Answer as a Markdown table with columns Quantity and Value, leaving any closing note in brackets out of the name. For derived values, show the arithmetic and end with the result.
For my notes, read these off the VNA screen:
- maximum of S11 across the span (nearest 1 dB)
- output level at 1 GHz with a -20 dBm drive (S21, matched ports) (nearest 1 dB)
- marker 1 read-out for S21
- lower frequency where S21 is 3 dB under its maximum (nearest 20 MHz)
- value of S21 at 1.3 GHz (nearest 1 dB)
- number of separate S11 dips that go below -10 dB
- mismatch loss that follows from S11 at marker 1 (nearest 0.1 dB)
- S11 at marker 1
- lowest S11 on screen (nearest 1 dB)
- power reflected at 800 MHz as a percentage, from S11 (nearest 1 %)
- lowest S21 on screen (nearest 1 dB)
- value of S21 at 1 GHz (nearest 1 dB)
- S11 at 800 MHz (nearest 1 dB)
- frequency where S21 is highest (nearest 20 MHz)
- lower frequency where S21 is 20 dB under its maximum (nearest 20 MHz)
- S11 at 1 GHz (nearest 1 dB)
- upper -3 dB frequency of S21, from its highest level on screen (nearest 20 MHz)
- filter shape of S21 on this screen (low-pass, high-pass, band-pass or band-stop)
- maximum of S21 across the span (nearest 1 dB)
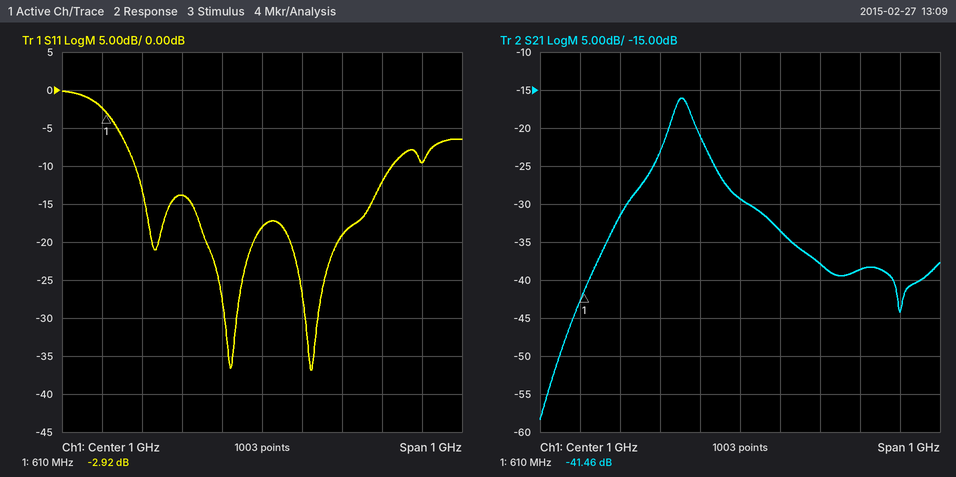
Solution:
| Quantity | Value |
|---|---|
| maximum of S11 across the span | 0 dB |
| output level at 1 GHz with a -20 dBm drive (S21, matched ports) | -20 dBm + (-29 dB) = -49 dBm |
| marker 1 read-out for S21 | -41.46 dB |
| lower frequency where S21 is 3 dB under its maximum | 820 MHz |
| value of S21 at 1.3 GHz | -39 dB |
| number of separate S11 dips that go below -10 dB | 3 |
| mismatch loss that follows from S11 at marker 1 | −10 log10(1 − 10^(-2.92/10)) ≈ 3.1 dB |
| S11 at marker 1 | -2.92 dB |
| lowest S11 on screen | -37 dB |
| power reflected at 800 MHz as a percentage, from S11 | 10^(-14/10) ≈ 4 % |
| lowest S21 on screen | -58 dB |
| value of S21 at 1 GHz | -29 dB |
| S11 at 800 MHz | -14 dB |
| frequency where S21 is highest | 860 MHz |
| lower frequency where S21 is 20 dB under its maximum | 660 MHz |
| S11 at 1 GHz | -18 dB |
| upper -3 dB frequency of S21, from its highest level on screen | 880 MHz |
| filter shape of S21 on this screen | band-pass |
| maximum of S21 across the span | -16 dB |
